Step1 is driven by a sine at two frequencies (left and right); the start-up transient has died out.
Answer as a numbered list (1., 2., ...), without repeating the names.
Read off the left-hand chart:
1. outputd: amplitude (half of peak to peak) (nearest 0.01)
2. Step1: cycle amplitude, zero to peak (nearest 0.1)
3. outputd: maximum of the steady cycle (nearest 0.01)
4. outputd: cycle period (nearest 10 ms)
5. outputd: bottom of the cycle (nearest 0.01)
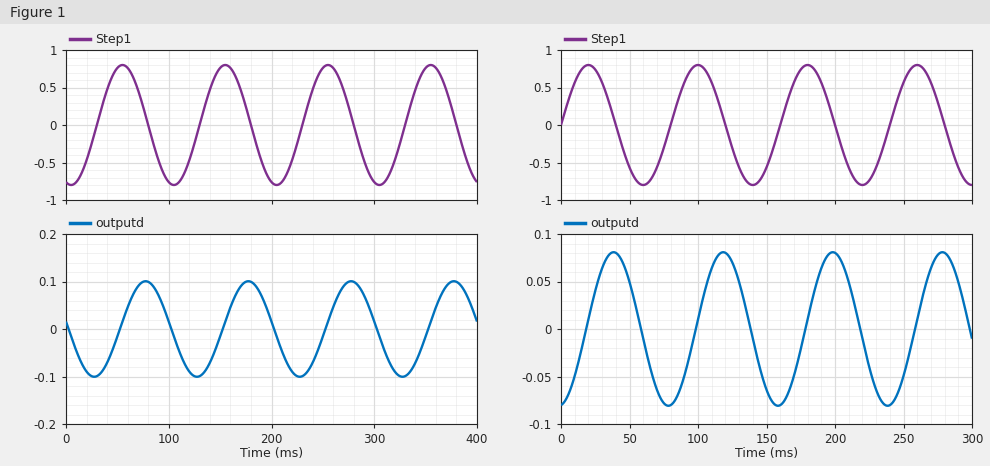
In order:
1. 0.10
2. 0.8
3. 0.10
4. 100 ms
5. -0.10
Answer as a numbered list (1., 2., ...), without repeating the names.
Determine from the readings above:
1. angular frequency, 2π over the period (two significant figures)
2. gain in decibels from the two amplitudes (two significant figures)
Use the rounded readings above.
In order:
1. 0.063 rad/ms
2. -18 dB
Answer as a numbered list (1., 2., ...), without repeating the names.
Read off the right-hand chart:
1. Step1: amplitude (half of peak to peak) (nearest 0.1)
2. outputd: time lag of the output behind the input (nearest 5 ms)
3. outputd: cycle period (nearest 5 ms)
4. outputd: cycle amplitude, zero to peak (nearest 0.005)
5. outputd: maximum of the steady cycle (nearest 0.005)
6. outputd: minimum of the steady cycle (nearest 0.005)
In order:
1. 0.8
2. 20 ms
3. 80 ms
4. 0.080
5. 0.080
6. -0.080
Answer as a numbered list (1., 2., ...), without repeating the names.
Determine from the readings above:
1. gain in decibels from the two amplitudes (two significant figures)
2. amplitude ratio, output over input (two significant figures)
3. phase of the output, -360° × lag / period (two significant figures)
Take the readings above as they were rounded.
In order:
1. -20 dB
2. 0.10
3. -90°
